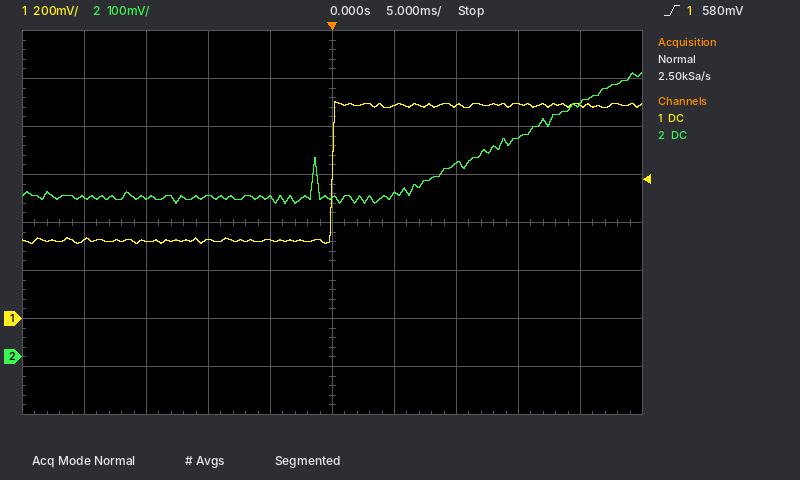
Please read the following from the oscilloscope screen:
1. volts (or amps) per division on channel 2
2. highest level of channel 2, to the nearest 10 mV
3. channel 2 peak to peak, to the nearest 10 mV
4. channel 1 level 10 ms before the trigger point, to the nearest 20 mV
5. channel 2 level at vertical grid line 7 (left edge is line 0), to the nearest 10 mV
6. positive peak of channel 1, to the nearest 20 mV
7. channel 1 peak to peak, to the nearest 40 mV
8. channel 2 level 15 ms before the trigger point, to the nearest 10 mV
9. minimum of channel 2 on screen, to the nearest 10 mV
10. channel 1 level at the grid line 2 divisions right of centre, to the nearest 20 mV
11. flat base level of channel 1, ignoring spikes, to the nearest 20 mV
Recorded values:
100 mV
590 mV
270 mV
320 mV
400 mV
900 mV
600 mV
330 mV
320 mV
880 mV
320 mV
